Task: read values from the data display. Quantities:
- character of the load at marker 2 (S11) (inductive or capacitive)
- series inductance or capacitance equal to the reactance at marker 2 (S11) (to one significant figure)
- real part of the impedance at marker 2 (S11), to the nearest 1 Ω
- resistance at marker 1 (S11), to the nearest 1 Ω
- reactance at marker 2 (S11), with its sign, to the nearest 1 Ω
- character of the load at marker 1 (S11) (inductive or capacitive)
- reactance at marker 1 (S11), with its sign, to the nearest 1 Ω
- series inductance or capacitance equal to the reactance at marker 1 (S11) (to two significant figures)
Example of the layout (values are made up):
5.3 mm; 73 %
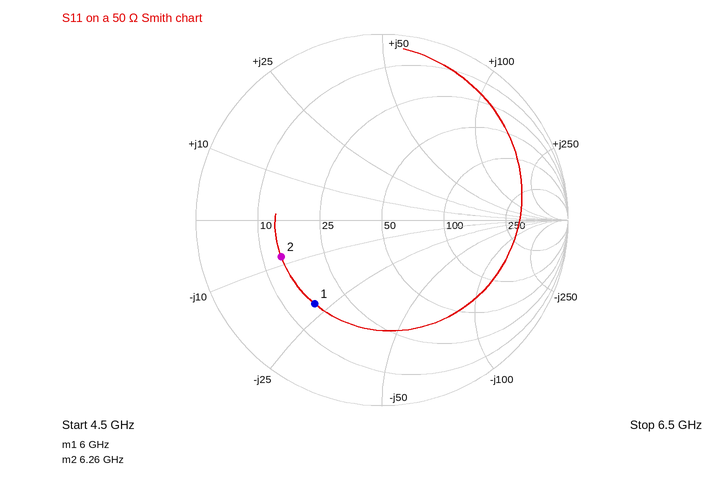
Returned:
capacitive; 3 pF; 14 Ω; 16 Ω; -8 Ω; capacitive; -22 Ω; 1.2 pF
